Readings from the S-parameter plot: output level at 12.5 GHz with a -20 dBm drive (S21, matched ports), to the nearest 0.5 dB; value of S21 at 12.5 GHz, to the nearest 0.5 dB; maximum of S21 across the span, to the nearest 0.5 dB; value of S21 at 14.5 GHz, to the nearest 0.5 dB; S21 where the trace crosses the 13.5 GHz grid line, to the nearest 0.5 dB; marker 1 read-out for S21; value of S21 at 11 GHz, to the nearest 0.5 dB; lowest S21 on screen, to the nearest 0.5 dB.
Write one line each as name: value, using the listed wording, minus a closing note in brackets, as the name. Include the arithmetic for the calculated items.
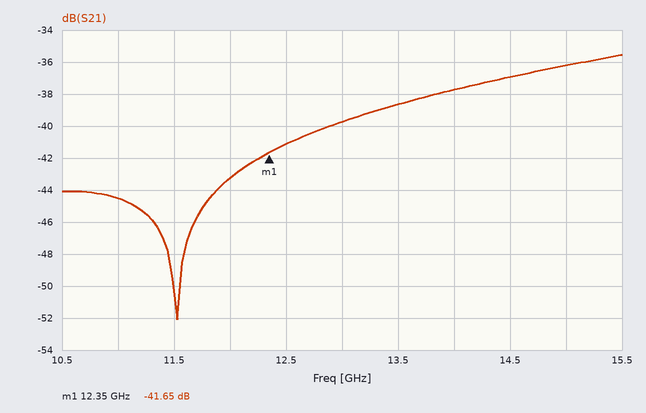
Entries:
output level at 12.5 GHz with a -20 dBm drive (S21, matched ports), to the nearest 0.5 dB: -20 dBm + (-41.0 dB) = -61.0 dBm
value of S21 at 12.5 GHz, to the nearest 0.5 dB: -41.0 dB
maximum of S21 across the span, to the nearest 0.5 dB: -35.5 dB
value of S21 at 14.5 GHz, to the nearest 0.5 dB: -37.0 dB
S21 where the trace crosses the 13.5 GHz grid line, to the nearest 0.5 dB: -38.5 dB
marker 1 read-out for S21: -41.65 dB
value of S21 at 11 GHz, to the nearest 0.5 dB: -44.5 dB
lowest S21 on screen, to the nearest 0.5 dB: -52.0 dB
